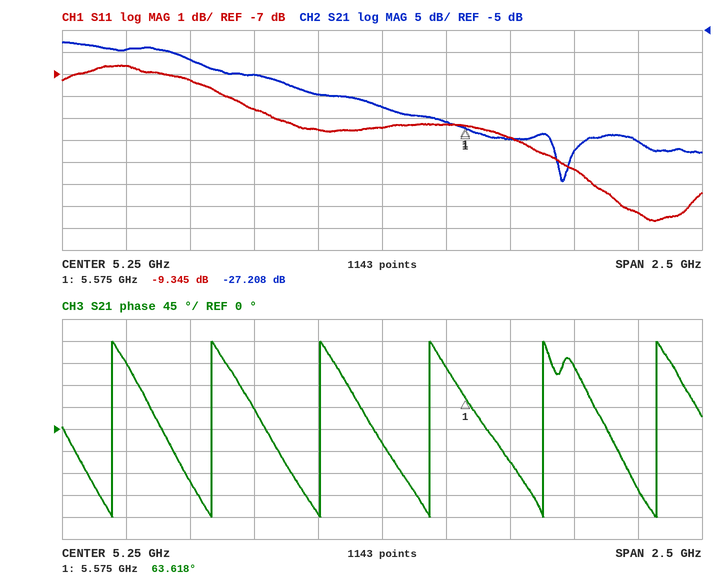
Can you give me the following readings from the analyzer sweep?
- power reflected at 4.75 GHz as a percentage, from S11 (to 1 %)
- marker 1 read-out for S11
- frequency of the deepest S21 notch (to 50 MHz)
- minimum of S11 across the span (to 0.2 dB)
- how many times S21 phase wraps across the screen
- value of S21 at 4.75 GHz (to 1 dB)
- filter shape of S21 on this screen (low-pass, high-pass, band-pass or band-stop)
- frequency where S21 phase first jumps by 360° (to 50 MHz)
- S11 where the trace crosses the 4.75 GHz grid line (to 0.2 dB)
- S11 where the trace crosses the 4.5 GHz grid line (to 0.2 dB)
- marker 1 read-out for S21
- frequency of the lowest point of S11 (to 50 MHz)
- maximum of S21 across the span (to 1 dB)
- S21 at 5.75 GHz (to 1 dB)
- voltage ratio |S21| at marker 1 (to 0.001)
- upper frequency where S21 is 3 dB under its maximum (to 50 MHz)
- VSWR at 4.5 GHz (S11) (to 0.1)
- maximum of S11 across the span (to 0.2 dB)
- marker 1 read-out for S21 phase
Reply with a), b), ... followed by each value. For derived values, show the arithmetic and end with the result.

a) 10^(-8.6/10) ≈ 14 %
b) -9.345 dB
c) 5.95 GHz
d) -13.6 dB
e) 6
f) -15 dB
g) low-pass
h) 4.20 GHz
i) -8.6 dB
j) -7.2 dB
k) -27.208 dB
l) 6.30 GHz
m) -8 dB
n) -30 dB
o) 10^(-27.208/20) ≈ 0.044
p) 4.45 GHz
q) |Γ| = 10^(-7.2/20) = 0.4365; VSWR = (1 + 0.4365)/(1 − 0.4365) ≈ 2.5
r) -6.6 dB
s) 63.618°
